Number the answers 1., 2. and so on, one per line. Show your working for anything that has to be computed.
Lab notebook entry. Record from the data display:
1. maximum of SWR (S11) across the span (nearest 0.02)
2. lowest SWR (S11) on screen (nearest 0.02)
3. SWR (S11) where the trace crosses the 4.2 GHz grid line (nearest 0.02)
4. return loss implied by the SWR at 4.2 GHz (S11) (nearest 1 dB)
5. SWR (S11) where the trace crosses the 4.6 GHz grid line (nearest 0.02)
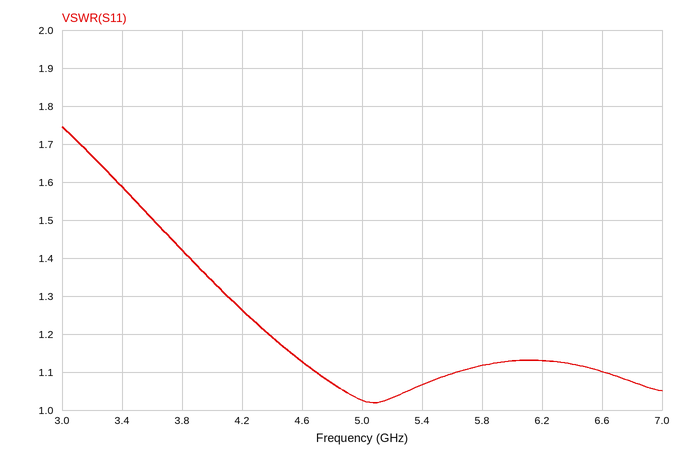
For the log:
1. 1.74
2. 1.02
3. 1.26
4. −20 log10((1.26 − 1)/(1.26 + 1)) ≈ 19 dB
5. 1.12
